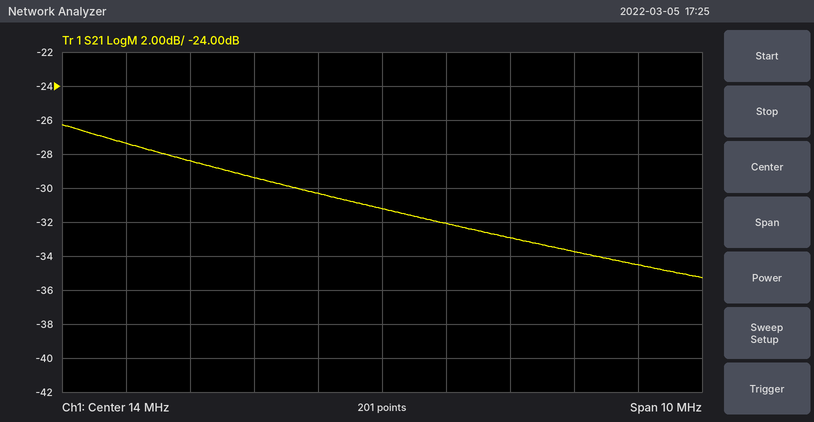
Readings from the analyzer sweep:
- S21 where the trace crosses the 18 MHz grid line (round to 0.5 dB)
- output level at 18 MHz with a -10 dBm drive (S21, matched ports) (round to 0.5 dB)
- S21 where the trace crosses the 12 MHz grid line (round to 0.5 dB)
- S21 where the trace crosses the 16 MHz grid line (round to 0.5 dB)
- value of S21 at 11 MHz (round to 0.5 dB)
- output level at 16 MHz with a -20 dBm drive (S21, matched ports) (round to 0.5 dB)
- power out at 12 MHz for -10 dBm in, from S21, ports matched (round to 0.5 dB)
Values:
-34.5 dB
-44.5 dBm
-29.5 dB
-33.0 dB
-28.5 dB
-53.0 dBm
-39.5 dBm
